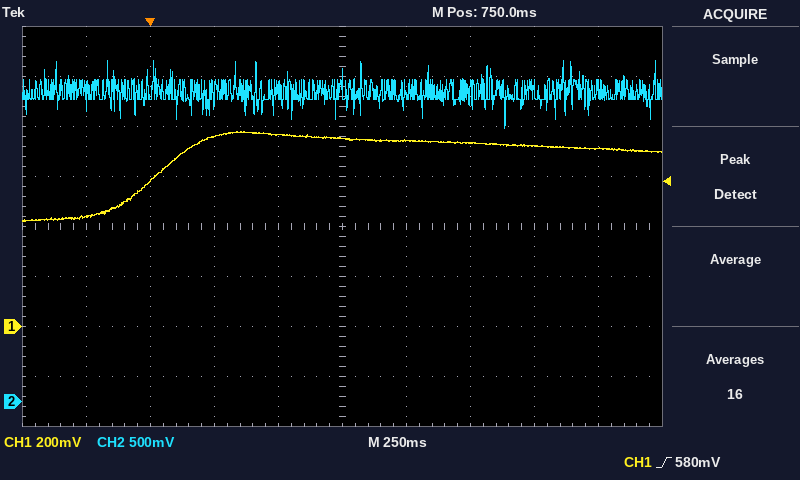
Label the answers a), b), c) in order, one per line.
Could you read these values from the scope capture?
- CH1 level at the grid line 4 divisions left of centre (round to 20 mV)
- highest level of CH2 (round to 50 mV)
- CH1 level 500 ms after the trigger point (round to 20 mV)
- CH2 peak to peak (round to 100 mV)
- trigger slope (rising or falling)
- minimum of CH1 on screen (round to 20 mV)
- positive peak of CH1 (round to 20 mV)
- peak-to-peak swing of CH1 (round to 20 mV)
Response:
a) 440 mV
b) 3.40 V
c) 760 mV
d) 700 mV
e) rising
f) 420 mV
g) 780 mV
h) 360 mV
